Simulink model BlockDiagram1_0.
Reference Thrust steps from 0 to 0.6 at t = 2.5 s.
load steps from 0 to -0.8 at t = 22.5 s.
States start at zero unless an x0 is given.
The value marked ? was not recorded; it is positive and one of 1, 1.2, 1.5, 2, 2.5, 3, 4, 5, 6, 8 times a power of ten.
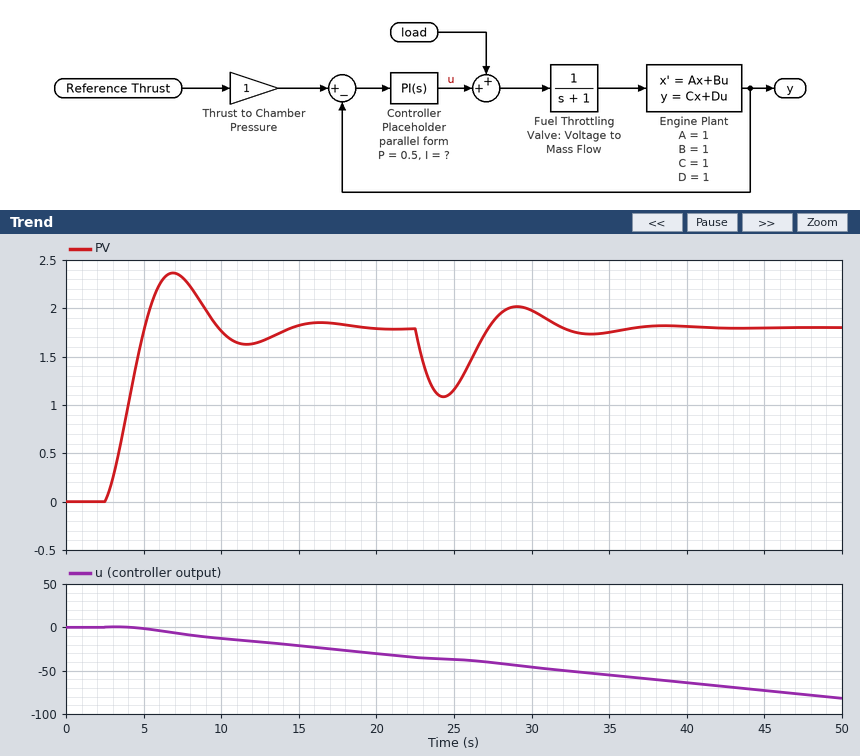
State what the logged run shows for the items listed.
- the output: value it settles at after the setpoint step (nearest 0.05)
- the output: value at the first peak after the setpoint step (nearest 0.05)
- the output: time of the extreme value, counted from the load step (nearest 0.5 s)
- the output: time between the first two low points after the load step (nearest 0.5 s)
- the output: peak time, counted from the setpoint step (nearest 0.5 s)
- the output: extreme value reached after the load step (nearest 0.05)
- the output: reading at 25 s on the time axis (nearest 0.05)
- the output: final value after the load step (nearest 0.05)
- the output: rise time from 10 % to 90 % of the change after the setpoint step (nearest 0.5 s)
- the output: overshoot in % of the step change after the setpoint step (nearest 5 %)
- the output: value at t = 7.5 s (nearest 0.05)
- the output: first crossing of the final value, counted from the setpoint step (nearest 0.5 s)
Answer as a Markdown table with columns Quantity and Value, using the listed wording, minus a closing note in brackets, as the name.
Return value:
| Quantity | Value |
|---|---|
| the output: value it settles at after the setpoint step | 1.80 |
| the output: value at the first peak after the setpoint step | 2.35 |
| the output: time of the extreme value, counted from the load step | 2.0 s |
| the output: time between the first two low points after the load step | 9.5 s |
| the output: peak time, counted from the setpoint step | 4.5 s |
| the output: extreme value reached after the load step | 1.10 |
| the output: reading at 25 s on the time axis | 1.15 |
| the output: final value after the load step | 1.80 |
| the output: rise time from 10 % to 90 % of the change after the setpoint step | 2.0 s |
| the output: overshoot in % of the step change after the setpoint step | 30 % |
| the output: value at t = 7.5 s | 2.30 |
| the output: first crossing of the final value, counted from the setpoint step | 2.5 s |
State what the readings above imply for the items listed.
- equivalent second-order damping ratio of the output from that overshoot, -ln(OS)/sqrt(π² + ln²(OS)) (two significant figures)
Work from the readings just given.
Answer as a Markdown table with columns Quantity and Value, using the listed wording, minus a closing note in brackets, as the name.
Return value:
| Quantity | Value |
|---|---|
| equivalent second-order damping ratio of the output from that overshoot, -ln(OS)/sqrt(π² + ln²(OS)) | 0.36 |
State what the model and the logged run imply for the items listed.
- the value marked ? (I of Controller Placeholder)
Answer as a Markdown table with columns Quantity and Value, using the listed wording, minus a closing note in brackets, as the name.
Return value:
| Quantity | Value |
|---|---|
| the value marked ? | 1.5 |
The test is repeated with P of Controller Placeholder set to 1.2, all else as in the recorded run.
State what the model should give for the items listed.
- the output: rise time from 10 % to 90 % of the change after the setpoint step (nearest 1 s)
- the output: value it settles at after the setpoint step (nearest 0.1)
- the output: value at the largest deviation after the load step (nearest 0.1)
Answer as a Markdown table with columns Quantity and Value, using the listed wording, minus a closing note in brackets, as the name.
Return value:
| Quantity | Value |
|---|---|
| the output: rise time from 10 % to 90 % of the change after the setpoint step | 3 s |
| the output: value it settles at after the setpoint step | 1.8 |
| the output: value at the largest deviation after the load step | 1.3 |
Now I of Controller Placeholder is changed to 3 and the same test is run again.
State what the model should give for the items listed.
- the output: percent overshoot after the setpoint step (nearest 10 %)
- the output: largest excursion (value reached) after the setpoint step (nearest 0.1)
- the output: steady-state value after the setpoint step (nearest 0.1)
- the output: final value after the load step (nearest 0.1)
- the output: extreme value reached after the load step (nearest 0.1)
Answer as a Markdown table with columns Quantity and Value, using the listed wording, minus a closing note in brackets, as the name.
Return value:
| Quantity | Value |
|---|---|
| the output: percent overshoot after the setpoint step | 60 % |
| the output: largest excursion (value reached) after the setpoint step | 1.4 |
| the output: steady-state value after the setpoint step | 0.9 |
| the output: final value after the load step | 0.9 |
| the output: extreme value reached after the load step | 0.5 |
